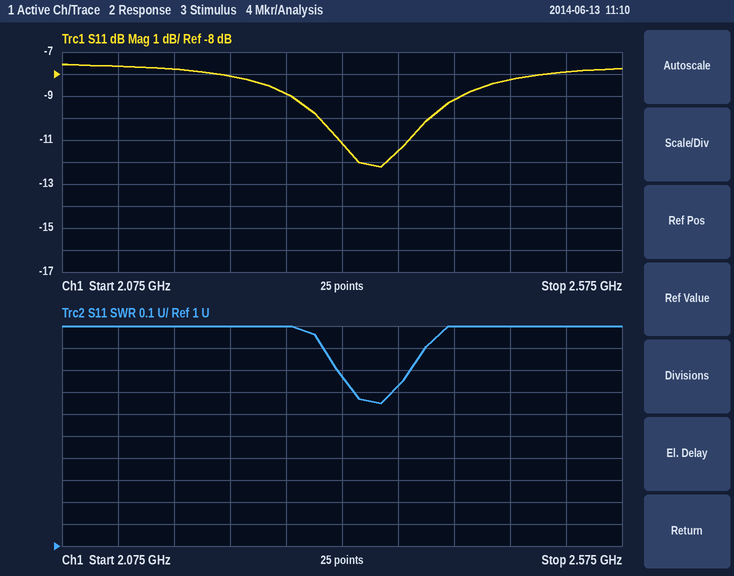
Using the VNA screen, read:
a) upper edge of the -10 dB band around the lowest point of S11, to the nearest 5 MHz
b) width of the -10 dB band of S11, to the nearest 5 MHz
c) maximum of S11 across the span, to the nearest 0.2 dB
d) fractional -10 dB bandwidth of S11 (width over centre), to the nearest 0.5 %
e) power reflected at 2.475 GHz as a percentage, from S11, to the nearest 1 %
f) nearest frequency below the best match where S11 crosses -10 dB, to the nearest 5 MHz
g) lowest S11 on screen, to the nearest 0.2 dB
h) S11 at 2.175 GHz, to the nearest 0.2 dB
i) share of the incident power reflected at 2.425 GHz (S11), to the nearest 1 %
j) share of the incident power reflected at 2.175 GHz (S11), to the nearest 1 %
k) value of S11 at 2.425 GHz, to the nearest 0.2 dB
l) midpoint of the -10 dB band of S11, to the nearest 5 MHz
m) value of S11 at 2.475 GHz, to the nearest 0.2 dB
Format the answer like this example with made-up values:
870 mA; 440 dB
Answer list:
2.405 GHz; 100 MHz; -7.6 dB; 4.0 %; 15 %; 2.305 GHz; -12.2 dB; -7.8 dB; 12 %; 17 %; -9.2 dB; 2.355 GHz; -8.2 dB
